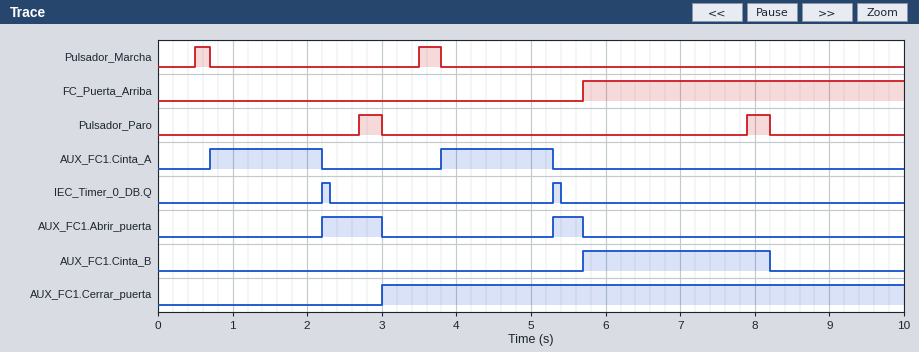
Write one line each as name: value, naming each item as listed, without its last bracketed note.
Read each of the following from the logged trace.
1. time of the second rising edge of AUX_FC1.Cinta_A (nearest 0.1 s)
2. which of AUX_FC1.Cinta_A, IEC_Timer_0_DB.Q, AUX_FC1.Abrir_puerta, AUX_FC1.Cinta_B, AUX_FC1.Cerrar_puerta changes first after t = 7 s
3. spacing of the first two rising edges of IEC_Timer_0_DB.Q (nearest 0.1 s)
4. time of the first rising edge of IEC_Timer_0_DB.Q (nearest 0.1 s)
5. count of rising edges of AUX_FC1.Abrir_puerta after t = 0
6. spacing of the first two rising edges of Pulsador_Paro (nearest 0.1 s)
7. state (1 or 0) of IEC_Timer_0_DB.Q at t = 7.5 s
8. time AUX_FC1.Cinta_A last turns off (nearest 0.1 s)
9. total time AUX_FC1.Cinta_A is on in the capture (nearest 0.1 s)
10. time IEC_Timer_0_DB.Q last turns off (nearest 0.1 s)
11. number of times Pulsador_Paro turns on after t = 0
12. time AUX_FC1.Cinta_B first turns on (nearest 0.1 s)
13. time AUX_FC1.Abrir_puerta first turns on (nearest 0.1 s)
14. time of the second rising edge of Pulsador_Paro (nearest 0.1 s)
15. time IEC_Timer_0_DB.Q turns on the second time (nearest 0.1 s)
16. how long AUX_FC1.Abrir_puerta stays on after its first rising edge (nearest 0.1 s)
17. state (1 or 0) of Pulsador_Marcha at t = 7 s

time of the second rising edge of AUX_FC1.Cinta_A: 3.8 s
which of AUX_FC1.Cinta_A, IEC_Timer_0_DB.Q, AUX_FC1.Abrir_puerta, AUX_FC1.Cinta_B, AUX_FC1.Cerrar_puerta changes first after t = 7 s: AUX_FC1.Cinta_B
spacing of the first two rising edges of IEC_Timer_0_DB.Q: 3.1 s
time of the first rising edge of IEC_Timer_0_DB.Q: 2.2 s
count of rising edges of AUX_FC1.Abrir_puerta after t = 0: 2
spacing of the first two rising edges of Pulsador_Paro: 5.2 s
state (1 or 0) of IEC_Timer_0_DB.Q at t = 7.5 s: 0
time AUX_FC1.Cinta_A last turns off: 5.3 s
total time AUX_FC1.Cinta_A is on in the capture: 3.0 s
time IEC_Timer_0_DB.Q last turns off: 5.4 s
number of times Pulsador_Paro turns on after t = 0: 2
time AUX_FC1.Cinta_B first turns on: 5.7 s
time AUX_FC1.Abrir_puerta first turns on: 2.2 s
time of the second rising edge of Pulsador_Paro: 7.9 s
time IEC_Timer_0_DB.Q turns on the second time: 5.3 s
how long AUX_FC1.Abrir_puerta stays on after its first rising edge: 0.8 s
state (1 or 0) of Pulsador_Marcha at t = 7 s: 0
